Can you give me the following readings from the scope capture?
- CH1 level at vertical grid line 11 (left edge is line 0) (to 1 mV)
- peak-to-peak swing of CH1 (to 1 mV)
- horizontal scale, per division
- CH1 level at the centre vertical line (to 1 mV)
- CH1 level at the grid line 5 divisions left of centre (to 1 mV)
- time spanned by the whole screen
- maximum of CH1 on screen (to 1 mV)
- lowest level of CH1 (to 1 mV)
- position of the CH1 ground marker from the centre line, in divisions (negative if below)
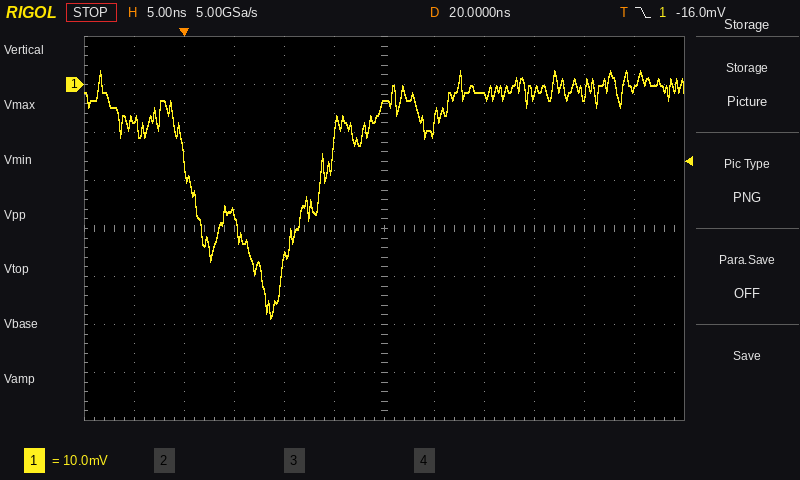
-1 mV
52 mV
5 ns
-4 mV
-7 mV
60 ns
3 mV
-49 mV
+3.0 div
